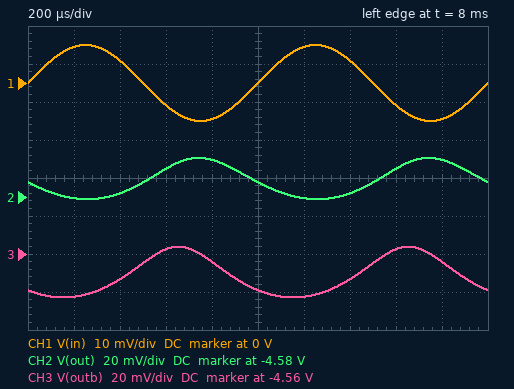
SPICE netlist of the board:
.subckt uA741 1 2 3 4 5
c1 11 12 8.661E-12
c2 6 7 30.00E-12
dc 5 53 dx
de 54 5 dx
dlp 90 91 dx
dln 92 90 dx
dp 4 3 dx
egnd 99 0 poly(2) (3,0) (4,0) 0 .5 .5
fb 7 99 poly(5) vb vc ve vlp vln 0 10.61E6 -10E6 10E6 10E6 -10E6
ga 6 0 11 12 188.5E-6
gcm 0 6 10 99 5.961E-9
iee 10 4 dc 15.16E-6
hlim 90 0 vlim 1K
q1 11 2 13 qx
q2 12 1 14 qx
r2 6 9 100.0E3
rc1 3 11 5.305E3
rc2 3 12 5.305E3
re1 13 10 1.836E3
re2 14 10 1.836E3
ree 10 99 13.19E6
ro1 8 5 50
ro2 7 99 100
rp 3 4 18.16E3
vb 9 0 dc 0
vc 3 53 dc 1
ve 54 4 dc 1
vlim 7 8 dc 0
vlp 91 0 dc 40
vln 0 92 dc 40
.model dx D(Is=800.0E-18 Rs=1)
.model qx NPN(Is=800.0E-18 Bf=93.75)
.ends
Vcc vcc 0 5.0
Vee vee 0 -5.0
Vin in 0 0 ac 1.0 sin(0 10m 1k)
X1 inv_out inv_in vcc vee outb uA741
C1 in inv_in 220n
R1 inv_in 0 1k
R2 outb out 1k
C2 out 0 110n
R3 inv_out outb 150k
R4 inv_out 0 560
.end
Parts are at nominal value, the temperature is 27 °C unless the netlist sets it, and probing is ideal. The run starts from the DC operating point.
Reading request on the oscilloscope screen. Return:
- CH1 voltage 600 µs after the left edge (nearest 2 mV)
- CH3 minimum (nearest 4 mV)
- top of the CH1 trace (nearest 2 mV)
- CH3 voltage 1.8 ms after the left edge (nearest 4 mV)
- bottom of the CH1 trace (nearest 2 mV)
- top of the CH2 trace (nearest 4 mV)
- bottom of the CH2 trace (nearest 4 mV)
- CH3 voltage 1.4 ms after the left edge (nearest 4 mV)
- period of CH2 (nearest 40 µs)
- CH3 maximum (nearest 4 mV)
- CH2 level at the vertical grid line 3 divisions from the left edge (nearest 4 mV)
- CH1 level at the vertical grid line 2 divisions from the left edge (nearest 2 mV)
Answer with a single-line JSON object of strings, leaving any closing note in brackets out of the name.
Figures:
{"CH1 voltage 600 µs after the left edge": "-6 mV", "CH3 minimum": "-4.584 V", "top of the CH1 trace": "10 mV", "CH3 voltage 1.8 ms after the left edge": "-4.564 V", "bottom of the CH1 trace": "-10 mV", "top of the CH2 trace": "-4.560 V", "bottom of the CH2 trace": "-4.580 V", "CH3 voltage 1.4 ms after the left edge": "-4.572 V", "period of CH2": "1.00 ms", "CH3 maximum": "-4.556 V", "CH2 level at the vertical grid line 3 divisions from the left edge": "-4.564 V", "CH1 level at the vertical grid line 2 divisions from the left edge": "6 mV"}
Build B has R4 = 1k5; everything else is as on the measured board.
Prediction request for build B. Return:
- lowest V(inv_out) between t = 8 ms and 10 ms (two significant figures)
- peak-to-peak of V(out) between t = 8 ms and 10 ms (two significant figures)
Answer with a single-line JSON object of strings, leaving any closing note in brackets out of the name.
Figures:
{"lowest V(inv_out) between t = 8 ms and 10 ms": "-46 mV", "peak-to-peak of V(out) between t = 8 ms and 10 ms": "6.6 mV"}
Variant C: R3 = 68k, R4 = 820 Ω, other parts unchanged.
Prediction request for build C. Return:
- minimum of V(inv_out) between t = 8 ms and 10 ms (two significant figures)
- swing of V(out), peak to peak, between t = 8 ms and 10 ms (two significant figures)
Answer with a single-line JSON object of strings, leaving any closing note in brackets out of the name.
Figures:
{"minimum of V(inv_out) between t = 8 ms and 10 ms": "-55 mV", "swing of V(out), peak to peak, between t = 8 ms and 10 ms": "5.0 mV"}
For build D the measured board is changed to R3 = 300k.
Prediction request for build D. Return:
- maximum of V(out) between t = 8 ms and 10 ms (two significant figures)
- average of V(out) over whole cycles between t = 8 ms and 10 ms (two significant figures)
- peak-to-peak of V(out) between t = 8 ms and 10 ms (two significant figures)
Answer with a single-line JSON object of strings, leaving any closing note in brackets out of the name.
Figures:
{"maximum of V(out) between t = 8 ms and 10 ms": "-4.5 V", "average of V(out) over whole cycles between t = 8 ms and 10 ms": "-4.5 V", "peak-to-peak of V(out) between t = 8 ms and 10 ms": "80 mV"}
